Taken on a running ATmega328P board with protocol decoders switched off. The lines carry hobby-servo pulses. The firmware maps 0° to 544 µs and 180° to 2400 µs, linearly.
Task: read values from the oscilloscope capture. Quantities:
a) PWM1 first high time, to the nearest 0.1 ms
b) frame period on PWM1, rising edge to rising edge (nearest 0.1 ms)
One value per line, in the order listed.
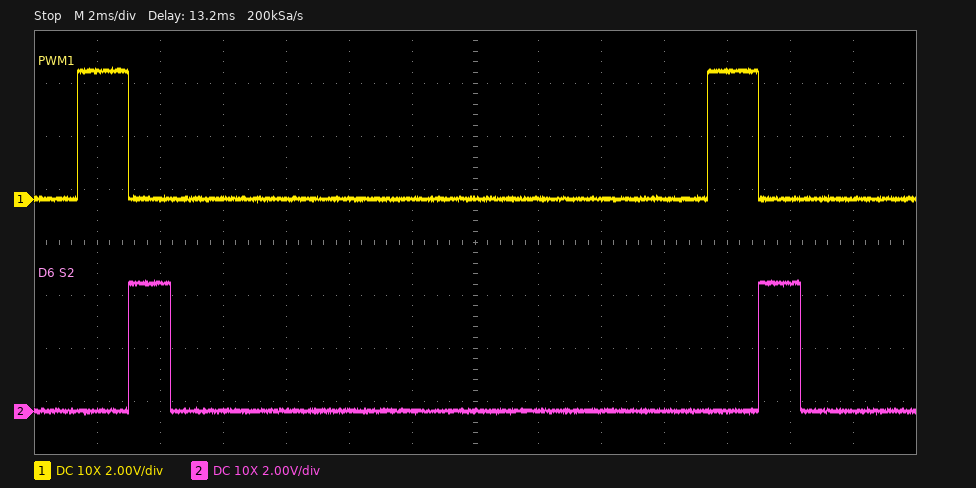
1.6 ms
20.0 ms
